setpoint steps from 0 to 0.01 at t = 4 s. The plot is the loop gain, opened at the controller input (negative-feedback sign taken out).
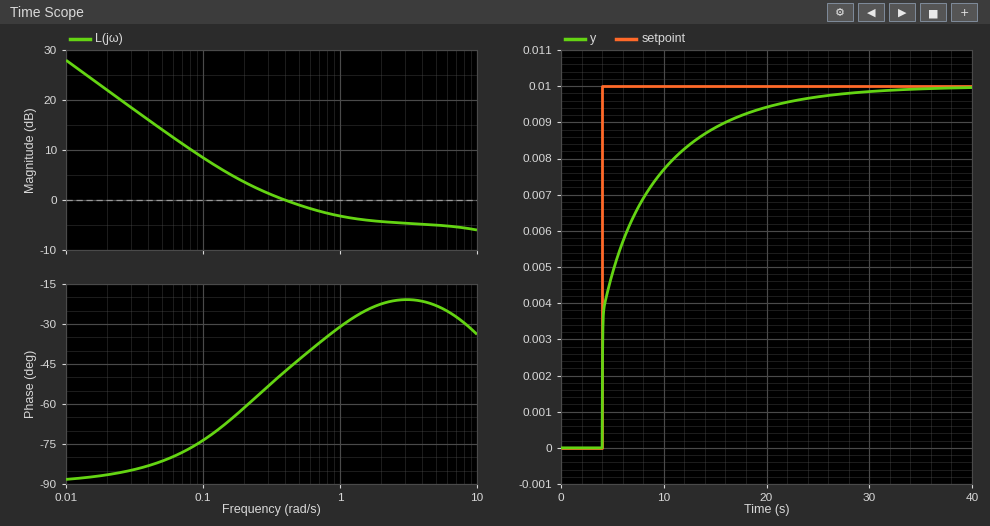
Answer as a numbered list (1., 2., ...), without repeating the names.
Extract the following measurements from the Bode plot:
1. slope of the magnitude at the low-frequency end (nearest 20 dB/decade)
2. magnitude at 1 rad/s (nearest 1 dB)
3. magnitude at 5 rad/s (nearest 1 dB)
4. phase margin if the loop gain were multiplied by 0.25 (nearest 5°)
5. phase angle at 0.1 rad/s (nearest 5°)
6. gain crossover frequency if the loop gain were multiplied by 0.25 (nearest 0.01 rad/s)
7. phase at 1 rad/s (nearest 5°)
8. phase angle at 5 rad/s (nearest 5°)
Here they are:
1. -20 dB/decade
2. -3 dB
3. -5 dB
4. 100°
5. -75°
6. 0.06 rad/s
7. -30°
8. -25°
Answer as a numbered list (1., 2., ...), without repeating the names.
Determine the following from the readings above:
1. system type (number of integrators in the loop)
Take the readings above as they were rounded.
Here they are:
1. 1
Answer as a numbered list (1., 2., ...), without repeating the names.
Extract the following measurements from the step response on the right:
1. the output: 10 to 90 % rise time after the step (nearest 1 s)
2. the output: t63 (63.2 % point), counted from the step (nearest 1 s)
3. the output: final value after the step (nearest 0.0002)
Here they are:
1. 12 s
2. 3 s
3. 0.0100
